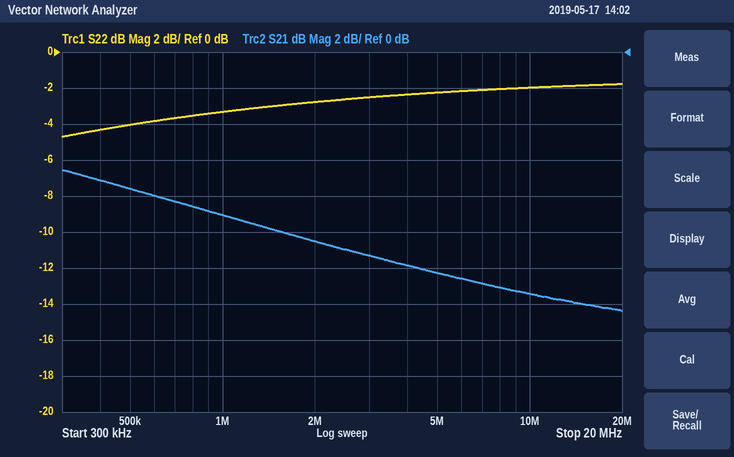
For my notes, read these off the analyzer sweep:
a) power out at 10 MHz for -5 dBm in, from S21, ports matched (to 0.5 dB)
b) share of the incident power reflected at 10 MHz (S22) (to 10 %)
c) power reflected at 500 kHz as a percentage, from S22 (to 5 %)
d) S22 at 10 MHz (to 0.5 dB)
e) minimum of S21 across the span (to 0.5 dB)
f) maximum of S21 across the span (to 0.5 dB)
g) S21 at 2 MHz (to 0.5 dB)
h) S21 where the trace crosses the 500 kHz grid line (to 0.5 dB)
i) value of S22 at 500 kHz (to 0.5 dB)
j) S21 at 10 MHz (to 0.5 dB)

-18.5 dBm
60 %
40 %
-2.0 dB
-14.5 dB
-6.5 dB
-10.5 dB
-7.5 dB
-4.0 dB
-13.5 dB
